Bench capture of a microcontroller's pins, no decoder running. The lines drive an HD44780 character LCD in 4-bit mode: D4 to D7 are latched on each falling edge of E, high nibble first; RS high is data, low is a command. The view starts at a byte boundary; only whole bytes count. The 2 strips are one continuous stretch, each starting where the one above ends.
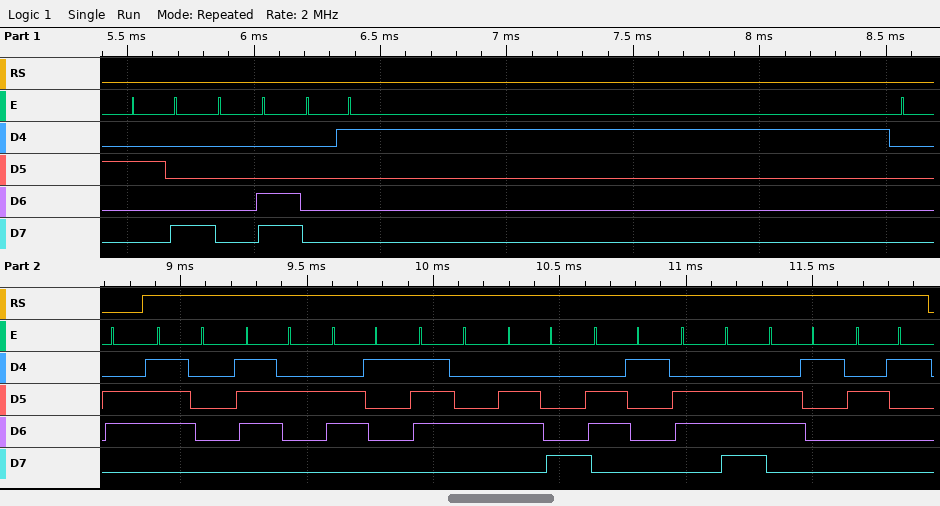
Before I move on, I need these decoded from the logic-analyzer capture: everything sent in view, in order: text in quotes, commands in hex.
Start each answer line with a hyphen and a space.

- 0x28 0x0C 0x01 0x06 "prathana!"
